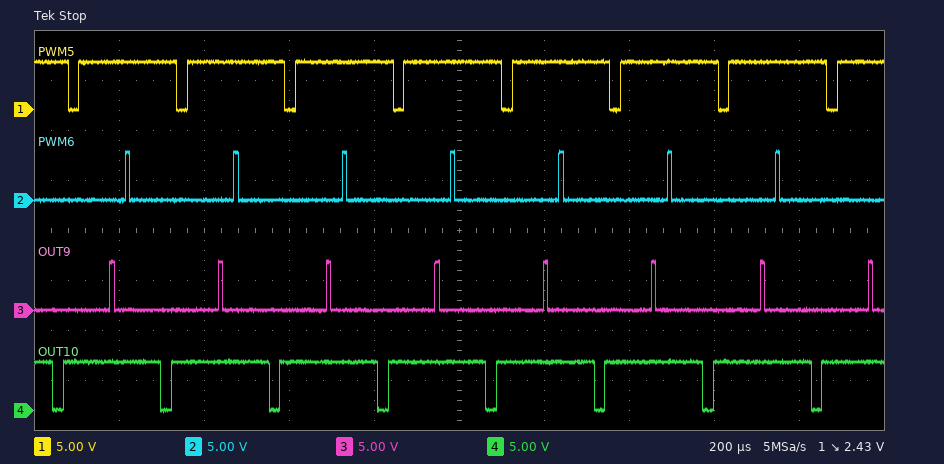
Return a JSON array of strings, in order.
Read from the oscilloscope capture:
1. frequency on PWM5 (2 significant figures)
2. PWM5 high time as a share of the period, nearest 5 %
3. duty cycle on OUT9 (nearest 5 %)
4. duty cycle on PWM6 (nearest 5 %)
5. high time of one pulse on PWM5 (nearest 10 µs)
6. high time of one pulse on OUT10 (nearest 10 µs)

["3.9 kHz", "90 %", "5 %", "5 %", "230 µs", "230 µs"]
